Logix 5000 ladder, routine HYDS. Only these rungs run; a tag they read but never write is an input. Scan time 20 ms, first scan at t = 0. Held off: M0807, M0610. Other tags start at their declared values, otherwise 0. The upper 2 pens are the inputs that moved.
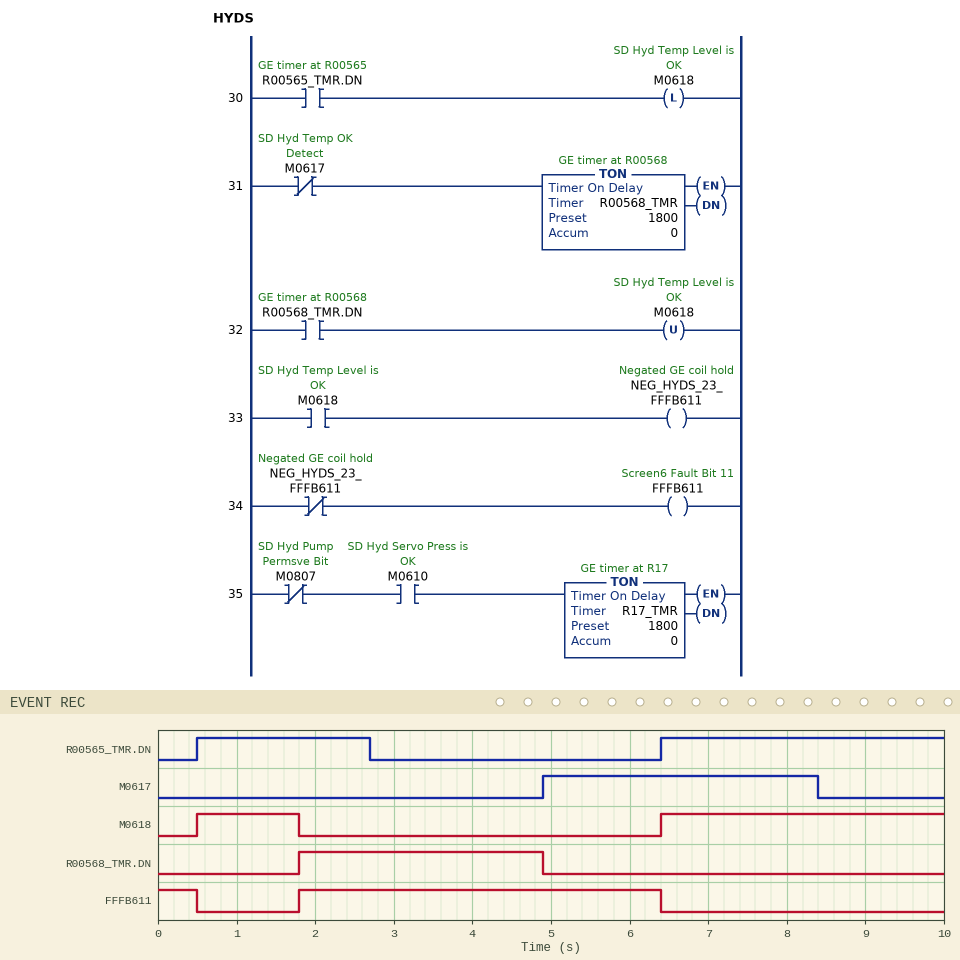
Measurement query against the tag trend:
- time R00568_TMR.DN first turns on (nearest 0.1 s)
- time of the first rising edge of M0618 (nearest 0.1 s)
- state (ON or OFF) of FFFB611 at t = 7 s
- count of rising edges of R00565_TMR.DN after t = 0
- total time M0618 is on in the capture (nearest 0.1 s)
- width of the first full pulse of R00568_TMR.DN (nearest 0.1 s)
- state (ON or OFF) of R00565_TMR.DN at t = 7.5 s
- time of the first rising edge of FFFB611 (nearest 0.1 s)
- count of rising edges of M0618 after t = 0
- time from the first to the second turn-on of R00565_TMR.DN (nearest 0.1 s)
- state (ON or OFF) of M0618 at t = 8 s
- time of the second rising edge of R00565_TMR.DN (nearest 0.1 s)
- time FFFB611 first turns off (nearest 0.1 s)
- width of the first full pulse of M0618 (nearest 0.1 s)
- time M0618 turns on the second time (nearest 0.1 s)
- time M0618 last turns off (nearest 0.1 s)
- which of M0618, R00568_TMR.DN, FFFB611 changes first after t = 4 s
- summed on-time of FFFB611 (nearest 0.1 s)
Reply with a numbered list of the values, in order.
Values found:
1. 1.8 s
2. 0.5 s
3. OFF
4. 2
5. 4.9 s
6. 3.1 s
7. ON
8. 1.8 s
9. 2
10. 5.9 s
11. ON
12. 6.4 s
13. 0.5 s
14. 1.3 s
15. 6.4 s
16. 1.8 s
17. R00568_TMR.DN
18. 5.1 s
